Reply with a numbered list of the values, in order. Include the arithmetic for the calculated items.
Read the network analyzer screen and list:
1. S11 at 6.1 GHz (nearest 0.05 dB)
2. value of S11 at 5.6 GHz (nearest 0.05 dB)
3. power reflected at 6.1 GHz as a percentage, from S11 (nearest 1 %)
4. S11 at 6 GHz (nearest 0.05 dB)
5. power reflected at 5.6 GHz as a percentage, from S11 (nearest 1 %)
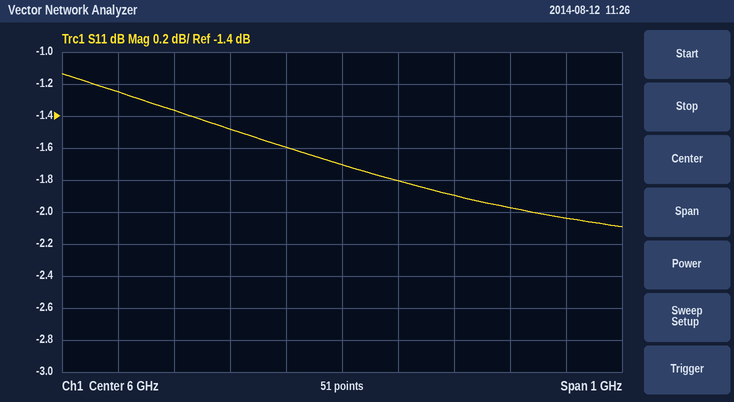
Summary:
1. -1.80 dB
2. -1.25 dB
3. 10^(-1.8/10) ≈ 66 %
4. -1.70 dB
5. 10^(-1.25/10) ≈ 75 %
